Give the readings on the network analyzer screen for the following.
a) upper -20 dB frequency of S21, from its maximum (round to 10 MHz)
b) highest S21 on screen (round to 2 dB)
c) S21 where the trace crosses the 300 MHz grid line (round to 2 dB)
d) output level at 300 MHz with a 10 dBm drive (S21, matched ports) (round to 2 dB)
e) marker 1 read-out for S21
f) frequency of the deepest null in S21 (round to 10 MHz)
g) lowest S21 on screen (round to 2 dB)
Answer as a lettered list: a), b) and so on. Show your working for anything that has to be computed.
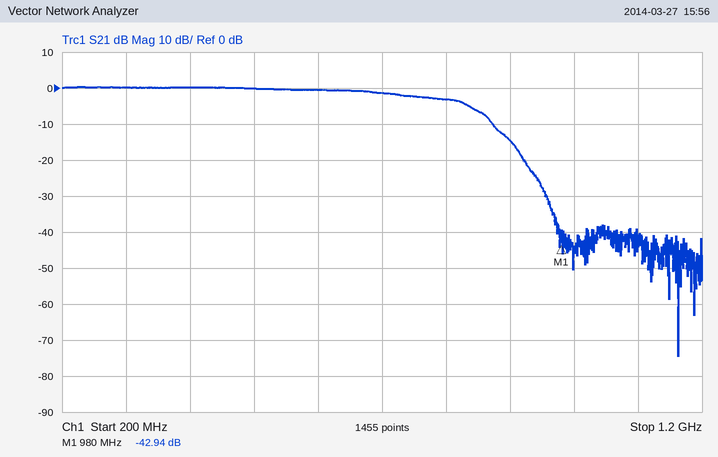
a) 920 MHz
b) 0 dB
c) 0 dB
d) 10 dBm + (0 dB) = 10 dBm
e) -42.94 dB
f) 1.16 GHz
g) -74 dB
